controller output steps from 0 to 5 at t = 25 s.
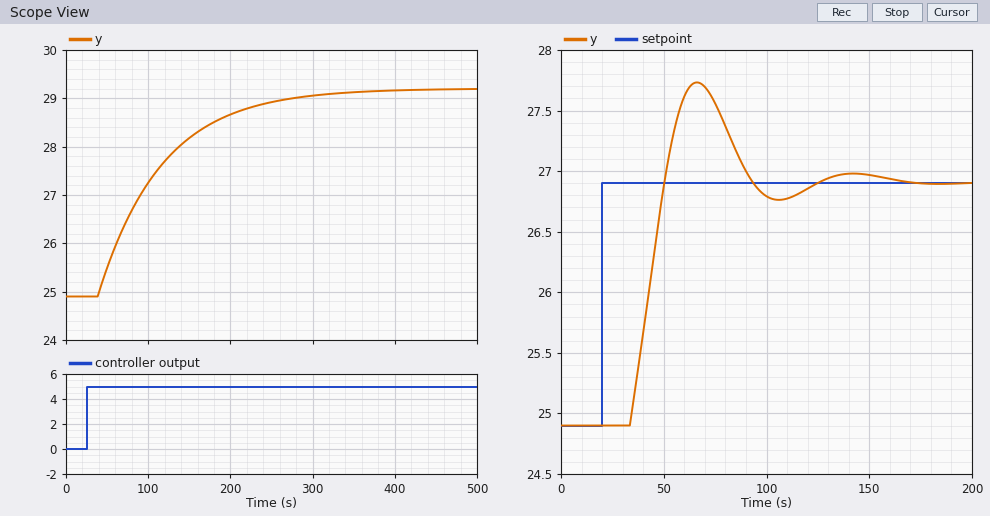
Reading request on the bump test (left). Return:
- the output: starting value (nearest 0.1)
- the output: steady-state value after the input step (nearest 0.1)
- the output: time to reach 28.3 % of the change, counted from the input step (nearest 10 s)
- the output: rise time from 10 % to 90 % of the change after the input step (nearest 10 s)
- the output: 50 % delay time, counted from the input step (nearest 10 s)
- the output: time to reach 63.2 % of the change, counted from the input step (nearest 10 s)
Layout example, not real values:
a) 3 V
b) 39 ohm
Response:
a) 24.9
b) 29.2
c) 40 s
d) 170 s
e) 70 s
f) 90 s
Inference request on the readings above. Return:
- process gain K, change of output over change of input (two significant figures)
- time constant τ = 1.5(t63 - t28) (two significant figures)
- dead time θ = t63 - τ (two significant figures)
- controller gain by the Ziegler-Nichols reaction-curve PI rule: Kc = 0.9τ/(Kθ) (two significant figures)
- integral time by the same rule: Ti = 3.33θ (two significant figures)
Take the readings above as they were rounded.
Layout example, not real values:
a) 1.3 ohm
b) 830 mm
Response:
a) 0.86
b) 75 s
c) 15 s
d) 5.2
e) 50 s
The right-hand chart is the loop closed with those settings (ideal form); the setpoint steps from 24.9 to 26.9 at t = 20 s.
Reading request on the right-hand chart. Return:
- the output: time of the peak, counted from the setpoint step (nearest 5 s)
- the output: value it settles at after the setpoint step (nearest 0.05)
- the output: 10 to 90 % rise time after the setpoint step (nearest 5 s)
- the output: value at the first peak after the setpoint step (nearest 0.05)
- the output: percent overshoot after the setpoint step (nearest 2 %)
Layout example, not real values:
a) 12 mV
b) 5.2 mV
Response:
a) 45 s
b) 26.90
c) 15 s
d) 27.75
e) 42 %
